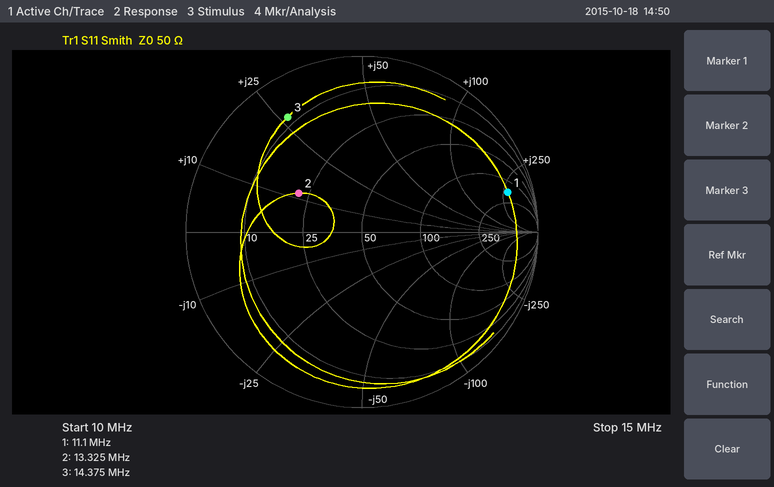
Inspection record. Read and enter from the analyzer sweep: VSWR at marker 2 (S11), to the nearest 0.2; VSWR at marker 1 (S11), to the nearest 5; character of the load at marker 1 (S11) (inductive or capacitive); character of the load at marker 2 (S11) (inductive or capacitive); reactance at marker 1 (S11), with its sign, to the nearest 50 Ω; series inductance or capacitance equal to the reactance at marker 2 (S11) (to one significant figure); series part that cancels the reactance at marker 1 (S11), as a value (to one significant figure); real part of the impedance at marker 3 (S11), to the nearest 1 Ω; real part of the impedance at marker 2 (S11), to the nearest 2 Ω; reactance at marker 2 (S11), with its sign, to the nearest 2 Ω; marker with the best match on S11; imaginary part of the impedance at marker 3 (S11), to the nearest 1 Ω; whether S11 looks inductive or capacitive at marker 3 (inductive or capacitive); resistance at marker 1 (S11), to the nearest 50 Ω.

2.4
15
inductive
inductive
+300 Ω
100 nH
50 pF
8 Ω
22 Ω
+12 Ω
marker 2
+27 Ω
inductive
150 Ω
